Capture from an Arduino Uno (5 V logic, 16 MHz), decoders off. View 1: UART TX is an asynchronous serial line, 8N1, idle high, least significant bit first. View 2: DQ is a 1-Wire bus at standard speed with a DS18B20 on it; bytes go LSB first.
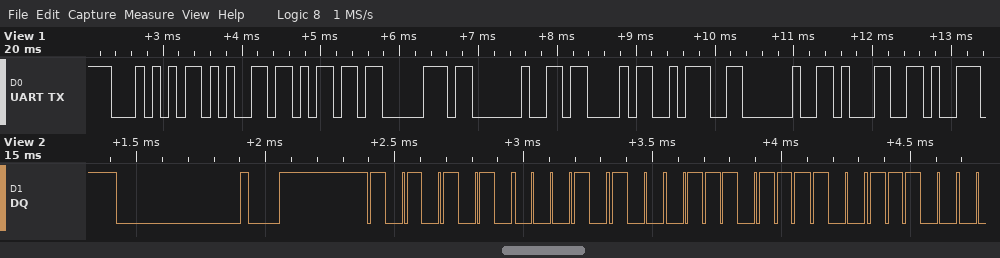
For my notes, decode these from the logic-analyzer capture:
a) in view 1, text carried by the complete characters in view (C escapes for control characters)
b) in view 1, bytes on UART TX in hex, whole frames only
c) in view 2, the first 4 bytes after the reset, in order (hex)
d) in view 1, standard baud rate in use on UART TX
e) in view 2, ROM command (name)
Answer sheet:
"Temp C: 1"
54 65 6D 70 20 43 3A 20 31
55 28 EE 39
9600 baud
Match ROM
